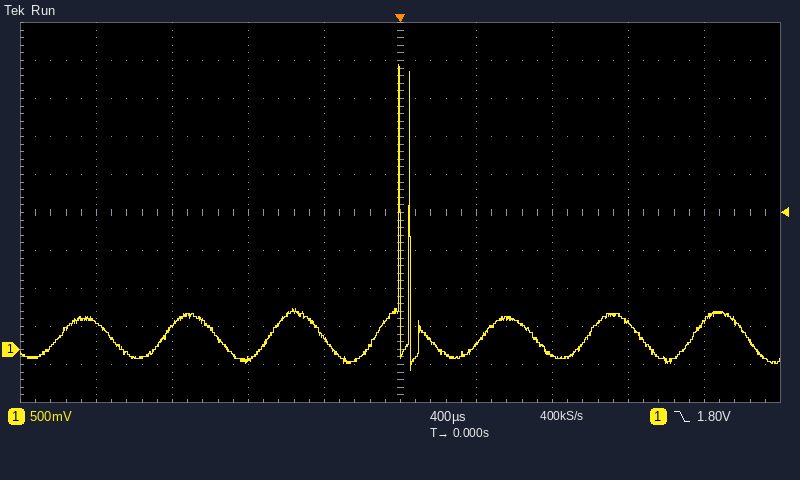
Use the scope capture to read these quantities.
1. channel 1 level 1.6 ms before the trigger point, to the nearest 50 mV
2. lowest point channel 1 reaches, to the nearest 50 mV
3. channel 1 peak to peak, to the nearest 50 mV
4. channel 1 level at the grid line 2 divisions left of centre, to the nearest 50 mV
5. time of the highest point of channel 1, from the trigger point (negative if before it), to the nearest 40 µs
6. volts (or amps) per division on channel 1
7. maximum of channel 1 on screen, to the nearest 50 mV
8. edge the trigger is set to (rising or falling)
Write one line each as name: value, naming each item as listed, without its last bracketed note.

channel 1 level 1.6 ms before the trigger point, to the nearest 50 mV: 350 mV
lowest point channel 1 reaches, to the nearest 50 mV: -300 mV
channel 1 peak to peak, to the nearest 50 mV: 4.05 V
channel 1 level at the grid line 2 divisions left of centre, to the nearest 50 mV: -150 mV
time of the highest point of channel 1, from the trigger point (negative if before it), to the nearest 40 µs: 0 µs
volts (or amps) per division on channel 1: 500 mV
maximum of channel 1 on screen, to the nearest 50 mV: 3.75 V
edge the trigger is set to: falling
